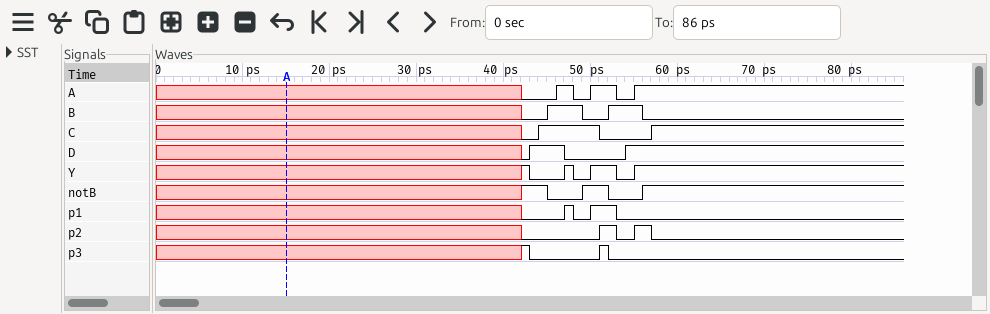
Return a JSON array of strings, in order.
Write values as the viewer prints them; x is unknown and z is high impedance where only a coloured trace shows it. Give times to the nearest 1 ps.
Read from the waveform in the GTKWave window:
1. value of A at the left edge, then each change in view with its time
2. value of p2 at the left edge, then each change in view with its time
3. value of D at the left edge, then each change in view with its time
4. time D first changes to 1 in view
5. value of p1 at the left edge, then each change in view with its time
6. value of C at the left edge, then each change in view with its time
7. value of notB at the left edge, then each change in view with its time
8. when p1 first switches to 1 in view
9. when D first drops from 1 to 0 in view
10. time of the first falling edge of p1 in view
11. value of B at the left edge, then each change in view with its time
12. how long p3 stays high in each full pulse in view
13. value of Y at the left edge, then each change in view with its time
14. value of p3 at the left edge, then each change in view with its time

["x, 0 at 42 ps, 1 at 46 ps, 0 at 48 ps, 1 at 50 ps, 0 at 53 ps, 1 at 55 ps", "x, 0 at 42 ps, 1 at 51 ps, 0 at 53 ps, 1 at 55 ps, 0 at 57 ps", "x, 0 at 42 ps, 1 at 43 ps, 0 at 47 ps, 1 at 54 ps", "43 ps", "x, 0 at 42 ps, 1 at 47 ps, 0 at 48 ps, 1 at 50 ps, 0 at 53 ps", "x, 0 at 42 ps, 1 at 44 ps, 0 at 51 ps, 1 at 57 ps", "x, 1 at 42 ps, 0 at 45 ps, 1 at 49 ps, 0 at 52 ps, 1 at 56 ps", "47 ps", "47 ps", "48 ps", "x, 0 at 42 ps, 1 at 45 ps, 0 at 49 ps, 1 at 52 ps, 0 at 56 ps", "1 ps", "x, 1 at 42 ps, 0 at 43 ps, 1 at 47 ps, 0 at 48 ps, 1 at 50 ps, 0 at 53 ps, 1 at 55 ps", "x, 1 at 42 ps, 0 at 43 ps, 1 at 51 ps, 0 at 52 ps"]
